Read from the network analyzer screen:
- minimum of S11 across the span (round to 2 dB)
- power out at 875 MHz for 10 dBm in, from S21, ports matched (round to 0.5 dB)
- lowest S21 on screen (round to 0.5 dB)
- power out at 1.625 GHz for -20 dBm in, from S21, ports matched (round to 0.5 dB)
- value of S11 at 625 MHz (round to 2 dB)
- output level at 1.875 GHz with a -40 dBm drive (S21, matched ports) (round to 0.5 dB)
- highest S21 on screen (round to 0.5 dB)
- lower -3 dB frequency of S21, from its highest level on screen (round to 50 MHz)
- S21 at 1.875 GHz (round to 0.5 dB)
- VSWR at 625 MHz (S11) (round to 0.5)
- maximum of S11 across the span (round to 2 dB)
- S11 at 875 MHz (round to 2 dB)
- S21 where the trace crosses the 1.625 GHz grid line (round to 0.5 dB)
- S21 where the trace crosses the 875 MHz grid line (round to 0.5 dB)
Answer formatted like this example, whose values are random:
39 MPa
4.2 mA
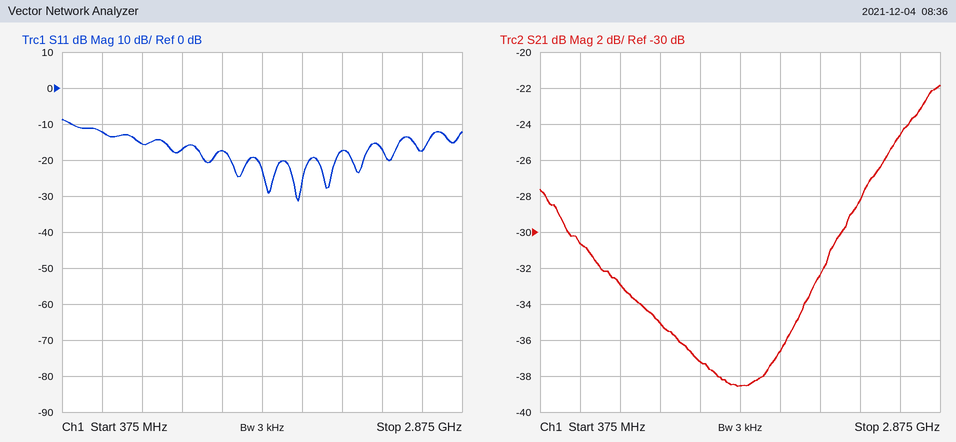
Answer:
-32 dB
-23.0 dBm
-38.5 dB
-58.5 dBm
-12 dB
-76.5 dBm
-22.0 dB
2.60 GHz
-36.5 dB
1.5
-8 dB
-16 dB
-38.5 dB
-33.0 dB
